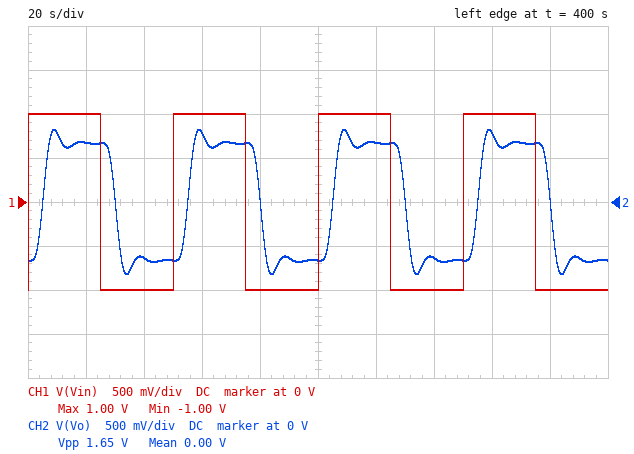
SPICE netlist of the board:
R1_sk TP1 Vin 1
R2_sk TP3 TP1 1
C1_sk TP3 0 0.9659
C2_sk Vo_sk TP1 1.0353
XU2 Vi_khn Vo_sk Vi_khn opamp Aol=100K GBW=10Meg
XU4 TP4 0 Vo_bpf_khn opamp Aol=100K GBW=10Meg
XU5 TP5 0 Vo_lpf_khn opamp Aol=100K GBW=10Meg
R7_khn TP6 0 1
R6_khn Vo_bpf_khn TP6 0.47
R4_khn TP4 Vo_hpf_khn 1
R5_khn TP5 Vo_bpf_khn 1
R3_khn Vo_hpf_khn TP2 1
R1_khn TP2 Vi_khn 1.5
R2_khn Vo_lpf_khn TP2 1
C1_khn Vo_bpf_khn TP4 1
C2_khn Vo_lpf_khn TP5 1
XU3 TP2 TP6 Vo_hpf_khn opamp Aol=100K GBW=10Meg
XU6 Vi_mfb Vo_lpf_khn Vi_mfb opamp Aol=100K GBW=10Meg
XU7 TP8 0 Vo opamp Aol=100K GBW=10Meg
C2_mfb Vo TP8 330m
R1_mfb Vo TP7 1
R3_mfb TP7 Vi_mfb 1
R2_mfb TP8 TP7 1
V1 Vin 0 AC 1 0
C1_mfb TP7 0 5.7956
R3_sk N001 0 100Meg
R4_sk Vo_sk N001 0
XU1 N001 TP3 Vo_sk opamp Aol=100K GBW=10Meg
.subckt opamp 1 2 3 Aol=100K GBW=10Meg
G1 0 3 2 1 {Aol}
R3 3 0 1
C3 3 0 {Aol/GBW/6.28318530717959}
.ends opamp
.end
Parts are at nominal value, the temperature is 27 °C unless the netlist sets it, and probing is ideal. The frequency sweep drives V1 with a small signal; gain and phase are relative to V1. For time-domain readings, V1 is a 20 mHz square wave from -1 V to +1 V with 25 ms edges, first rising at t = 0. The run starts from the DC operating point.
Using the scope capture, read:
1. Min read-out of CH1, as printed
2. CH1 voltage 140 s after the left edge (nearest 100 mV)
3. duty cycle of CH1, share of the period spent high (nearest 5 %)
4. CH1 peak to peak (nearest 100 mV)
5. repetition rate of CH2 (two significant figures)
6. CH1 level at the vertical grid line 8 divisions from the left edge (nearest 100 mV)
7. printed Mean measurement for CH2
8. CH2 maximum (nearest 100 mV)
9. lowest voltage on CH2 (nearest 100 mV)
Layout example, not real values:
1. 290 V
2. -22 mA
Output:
1. -1.00 V
2. -1.0 V
3. 50 %
4. 2.0 V
5. 20 mHz
6. 1.0 V
7. 0.00 V
8. 800 mV
9. -800 mV
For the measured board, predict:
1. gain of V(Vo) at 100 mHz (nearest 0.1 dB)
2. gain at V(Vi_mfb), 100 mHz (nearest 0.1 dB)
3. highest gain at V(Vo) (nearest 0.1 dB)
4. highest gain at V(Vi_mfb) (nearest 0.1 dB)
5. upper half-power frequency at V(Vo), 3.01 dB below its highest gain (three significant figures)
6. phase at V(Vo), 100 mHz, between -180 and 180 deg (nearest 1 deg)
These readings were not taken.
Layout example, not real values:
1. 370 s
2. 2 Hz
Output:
1. -4.9 dB
2. -8.4 dB
3. -3.5 dB
4. -3.5 dB
5. 113 mHz
6. 166 deg
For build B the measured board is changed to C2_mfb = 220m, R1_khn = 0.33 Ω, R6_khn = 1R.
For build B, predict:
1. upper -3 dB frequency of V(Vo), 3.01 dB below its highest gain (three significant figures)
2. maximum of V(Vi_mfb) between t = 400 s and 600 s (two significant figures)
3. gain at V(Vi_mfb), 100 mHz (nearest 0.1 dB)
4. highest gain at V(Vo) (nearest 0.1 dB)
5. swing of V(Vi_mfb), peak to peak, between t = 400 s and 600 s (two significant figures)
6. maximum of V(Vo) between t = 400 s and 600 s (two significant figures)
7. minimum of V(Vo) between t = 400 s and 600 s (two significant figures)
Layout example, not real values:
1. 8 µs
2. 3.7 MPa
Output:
1. 89.0 mHz
2. 3.0 V
3. 2.4 dB
4. 9.6 dB
5. 6.1 V
6. 3.1 V
7. -3.1 V
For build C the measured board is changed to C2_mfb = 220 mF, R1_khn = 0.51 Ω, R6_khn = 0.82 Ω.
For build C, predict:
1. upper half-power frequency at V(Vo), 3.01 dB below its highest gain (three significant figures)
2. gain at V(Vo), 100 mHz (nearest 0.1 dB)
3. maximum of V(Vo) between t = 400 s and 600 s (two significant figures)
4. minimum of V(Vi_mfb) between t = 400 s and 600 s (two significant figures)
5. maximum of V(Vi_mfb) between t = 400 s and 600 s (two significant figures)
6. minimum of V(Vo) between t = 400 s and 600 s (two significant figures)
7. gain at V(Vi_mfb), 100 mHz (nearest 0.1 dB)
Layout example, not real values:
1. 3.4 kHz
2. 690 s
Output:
1. 115 mHz
2. 3.5 dB
3. 2.1 V
4. -2.0 V
5. 2.0 V
6. -2.1 V
7. -0.3 dB
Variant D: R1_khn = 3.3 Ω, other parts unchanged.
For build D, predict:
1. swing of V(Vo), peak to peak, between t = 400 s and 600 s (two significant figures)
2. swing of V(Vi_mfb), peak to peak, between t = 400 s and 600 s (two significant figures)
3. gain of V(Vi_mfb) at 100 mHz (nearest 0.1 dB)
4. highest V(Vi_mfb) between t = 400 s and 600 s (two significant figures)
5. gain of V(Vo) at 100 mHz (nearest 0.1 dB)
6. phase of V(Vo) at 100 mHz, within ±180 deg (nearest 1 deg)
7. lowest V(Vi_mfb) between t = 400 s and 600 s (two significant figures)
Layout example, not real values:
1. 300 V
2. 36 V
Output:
1. 790 mV
2. 610 mV
3. -14.3 dB
4. 300 mV
5. -10.8 dB
6. 170 deg
7. -300 mV
